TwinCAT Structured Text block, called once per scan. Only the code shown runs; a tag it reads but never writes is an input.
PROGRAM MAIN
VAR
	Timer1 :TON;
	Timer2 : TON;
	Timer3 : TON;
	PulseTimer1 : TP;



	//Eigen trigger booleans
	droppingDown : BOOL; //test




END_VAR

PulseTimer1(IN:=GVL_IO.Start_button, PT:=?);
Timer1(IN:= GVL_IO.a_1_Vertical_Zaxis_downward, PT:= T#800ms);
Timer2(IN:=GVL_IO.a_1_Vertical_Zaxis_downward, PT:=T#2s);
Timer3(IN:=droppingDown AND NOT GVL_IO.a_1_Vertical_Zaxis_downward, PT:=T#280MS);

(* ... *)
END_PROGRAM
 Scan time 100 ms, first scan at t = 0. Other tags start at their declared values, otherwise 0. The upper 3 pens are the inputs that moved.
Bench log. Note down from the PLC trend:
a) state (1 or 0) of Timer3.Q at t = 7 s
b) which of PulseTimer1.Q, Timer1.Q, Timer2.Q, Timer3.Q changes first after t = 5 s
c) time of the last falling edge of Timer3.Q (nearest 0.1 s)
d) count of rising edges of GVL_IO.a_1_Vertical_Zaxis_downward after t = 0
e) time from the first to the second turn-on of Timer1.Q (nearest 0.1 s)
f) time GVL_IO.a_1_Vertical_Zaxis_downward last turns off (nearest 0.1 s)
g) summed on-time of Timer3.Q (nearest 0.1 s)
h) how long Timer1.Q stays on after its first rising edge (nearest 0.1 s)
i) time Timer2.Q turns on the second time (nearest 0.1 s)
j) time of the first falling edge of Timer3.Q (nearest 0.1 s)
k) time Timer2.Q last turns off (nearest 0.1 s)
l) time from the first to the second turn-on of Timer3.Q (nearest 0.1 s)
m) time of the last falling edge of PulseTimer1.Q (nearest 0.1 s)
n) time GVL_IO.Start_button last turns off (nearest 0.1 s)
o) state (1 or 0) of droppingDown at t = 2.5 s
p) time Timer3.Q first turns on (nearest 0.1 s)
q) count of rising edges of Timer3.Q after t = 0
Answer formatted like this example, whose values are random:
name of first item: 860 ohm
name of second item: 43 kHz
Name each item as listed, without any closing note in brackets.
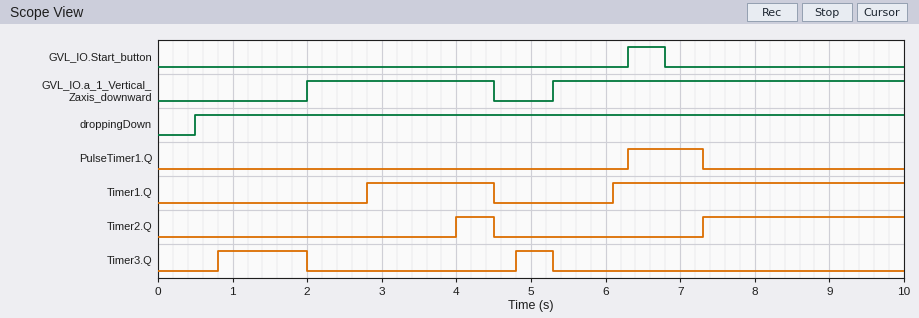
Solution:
state (1 or 0) of Timer3.Q at t = 7 s: 0
which of PulseTimer1.Q, Timer1.Q, Timer2.Q, Timer3.Q changes first after t = 5 s: Timer3.Q
time of the last falling edge of Timer3.Q: 5.3 s
count of rising edges of GVL_IO.a_1_Vertical_Zaxis_downward after t = 0: 2
time from the first to the second turn-on of Timer1.Q: 3.3 s
time GVL_IO.a_1_Vertical_Zaxis_downward last turns off: 4.5 s
summed on-time of Timer3.Q: 1.7 s
how long Timer1.Q stays on after its first rising edge: 1.7 s
time Timer2.Q turns on the second time: 7.3 s
time of the first falling edge of Timer3.Q: 2.0 s
time Timer2.Q last turns off: 4.5 s
time from the first to the second turn-on of Timer3.Q: 4.0 s
time of the last falling edge of PulseTimer1.Q: 7.3 s
time GVL_IO.Start_button last turns off: 6.8 s
state (1 or 0) of droppingDown at t = 2.5 s: 1
time Timer3.Q first turns on: 0.8 s
count of rising edges of Timer3.Q after t = 0: 2
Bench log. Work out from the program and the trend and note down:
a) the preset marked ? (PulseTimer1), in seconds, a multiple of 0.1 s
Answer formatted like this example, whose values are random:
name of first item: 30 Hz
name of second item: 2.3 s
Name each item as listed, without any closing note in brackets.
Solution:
the preset marked ? (PulseTimer1), in seconds, a multiple of 0.1 s: 1.0 s
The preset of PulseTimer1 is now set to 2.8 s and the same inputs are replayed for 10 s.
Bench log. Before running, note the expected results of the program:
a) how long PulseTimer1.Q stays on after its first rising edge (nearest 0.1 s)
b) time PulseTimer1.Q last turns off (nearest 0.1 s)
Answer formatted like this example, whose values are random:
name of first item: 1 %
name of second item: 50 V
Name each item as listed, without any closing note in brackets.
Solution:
how long PulseTimer1.Q stays on after its first rising edge: 2.8 s
time PulseTimer1.Q last turns off: 9.1 s
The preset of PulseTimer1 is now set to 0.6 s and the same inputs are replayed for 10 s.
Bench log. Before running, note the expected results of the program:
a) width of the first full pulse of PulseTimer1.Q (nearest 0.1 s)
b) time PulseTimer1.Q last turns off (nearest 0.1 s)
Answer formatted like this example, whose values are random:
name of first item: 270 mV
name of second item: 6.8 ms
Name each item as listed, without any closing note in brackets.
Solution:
width of the first full pulse of PulseTimer1.Q: 0.6 s
time PulseTimer1.Q last turns off: 6.9 s
